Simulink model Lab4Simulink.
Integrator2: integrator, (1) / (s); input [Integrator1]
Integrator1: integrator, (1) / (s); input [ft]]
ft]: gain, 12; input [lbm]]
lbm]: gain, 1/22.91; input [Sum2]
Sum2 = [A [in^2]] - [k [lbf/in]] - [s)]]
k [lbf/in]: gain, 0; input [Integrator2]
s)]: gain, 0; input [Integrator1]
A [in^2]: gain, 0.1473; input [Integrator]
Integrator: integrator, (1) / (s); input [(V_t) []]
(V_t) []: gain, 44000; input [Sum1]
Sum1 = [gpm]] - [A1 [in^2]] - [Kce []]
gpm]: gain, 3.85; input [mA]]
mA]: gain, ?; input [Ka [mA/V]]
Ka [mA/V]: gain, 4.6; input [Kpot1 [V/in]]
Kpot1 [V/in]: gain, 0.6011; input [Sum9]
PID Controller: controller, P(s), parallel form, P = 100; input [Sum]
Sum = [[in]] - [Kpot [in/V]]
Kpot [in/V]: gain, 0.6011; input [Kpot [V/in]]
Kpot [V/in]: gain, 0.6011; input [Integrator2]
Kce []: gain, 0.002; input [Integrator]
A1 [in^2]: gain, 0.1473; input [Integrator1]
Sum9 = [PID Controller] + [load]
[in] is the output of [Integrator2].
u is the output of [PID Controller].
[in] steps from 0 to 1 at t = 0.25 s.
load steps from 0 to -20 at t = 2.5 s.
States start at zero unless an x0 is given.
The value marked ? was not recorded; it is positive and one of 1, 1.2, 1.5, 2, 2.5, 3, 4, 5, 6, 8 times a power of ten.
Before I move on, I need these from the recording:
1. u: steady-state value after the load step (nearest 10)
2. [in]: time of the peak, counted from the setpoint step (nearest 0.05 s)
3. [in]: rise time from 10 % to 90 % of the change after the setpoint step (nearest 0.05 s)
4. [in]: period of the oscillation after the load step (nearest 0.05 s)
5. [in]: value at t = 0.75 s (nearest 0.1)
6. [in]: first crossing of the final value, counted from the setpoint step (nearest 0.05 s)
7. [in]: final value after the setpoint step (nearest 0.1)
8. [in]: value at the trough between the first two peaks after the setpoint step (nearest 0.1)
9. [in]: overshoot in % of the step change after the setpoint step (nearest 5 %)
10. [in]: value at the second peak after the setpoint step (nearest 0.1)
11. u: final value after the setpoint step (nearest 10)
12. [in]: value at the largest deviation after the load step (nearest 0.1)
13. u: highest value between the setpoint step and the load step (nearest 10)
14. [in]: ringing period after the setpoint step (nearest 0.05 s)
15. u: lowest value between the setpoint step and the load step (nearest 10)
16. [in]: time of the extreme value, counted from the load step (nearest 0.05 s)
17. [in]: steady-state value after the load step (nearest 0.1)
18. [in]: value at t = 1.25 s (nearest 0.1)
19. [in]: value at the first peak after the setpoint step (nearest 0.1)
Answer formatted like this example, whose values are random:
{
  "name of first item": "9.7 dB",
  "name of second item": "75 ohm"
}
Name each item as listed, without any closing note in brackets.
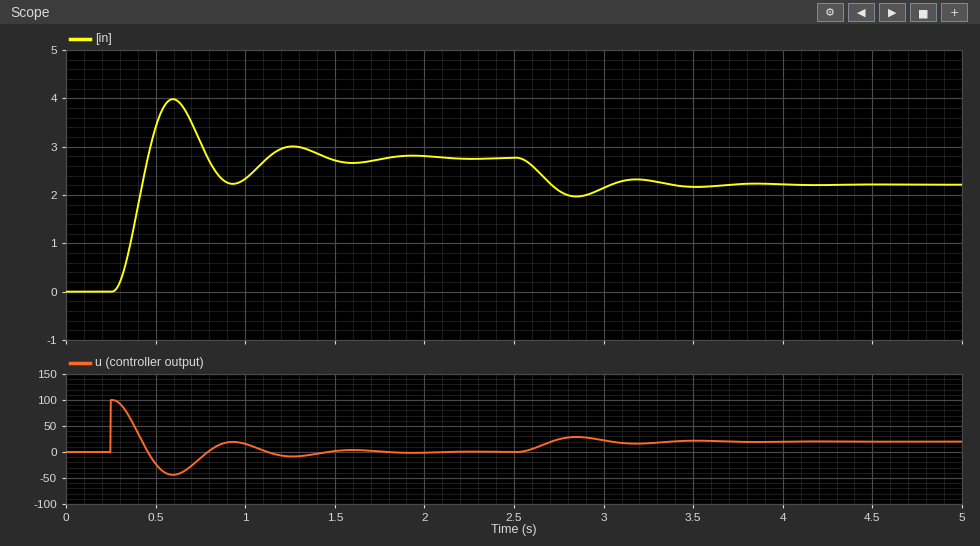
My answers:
{
  "u: steady-state value after the load step": "20",
  "[in]: time of the peak, counted from the setpoint step": "0.35 s",
  "[in]: rise time from 10 % to 90 % of the change after the setpoint step": "0.15 s",
  "[in]: period of the oscillation after the load step": "0.65 s",
  "[in]: value at t = 0.75 s": "3.1",
  "[in]: first crossing of the final value, counted from the setpoint step": "0.20 s",
  "[in]: final value after the setpoint step": "2.8",
  "[in]: value at the trough between the first two peaks after the setpoint step": "2.2",
  "[in]: overshoot in % of the step change after the setpoint step": "45 %",
  "[in]: value at the second peak after the setpoint step": "3.0",
  "u: final value after the setpoint step": "0",
  "[in]: value at the largest deviation after the load step": "2.0",
  "u: highest value between the setpoint step and the load step": "100",
  "[in]: ringing period after the setpoint step": "0.65 s",
  "u: lowest value between the setpoint step and the load step": "-40",
  "[in]: time of the extreme value, counted from the load step": "0.35 s",
  "[in]: steady-state value after the load step": "2.2",
  "[in]: value at t = 1.25 s": "3.0",
  "[in]: value at the first peak after the setpoint step": "4.0"
}
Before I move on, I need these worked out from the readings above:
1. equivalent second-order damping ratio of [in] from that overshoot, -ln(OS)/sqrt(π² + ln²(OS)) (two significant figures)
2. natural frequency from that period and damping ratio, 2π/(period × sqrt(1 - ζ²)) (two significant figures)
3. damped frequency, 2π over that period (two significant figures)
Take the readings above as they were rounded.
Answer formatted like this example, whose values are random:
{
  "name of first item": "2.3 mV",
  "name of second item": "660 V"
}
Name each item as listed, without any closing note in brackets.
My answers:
{
  "equivalent second-order damping ratio of [in] from that overshoot, -ln(OS)/sqrt(π² + ln²(OS))": "0.25",
  "natural frequency from that period and damping ratio, 2π/(period × sqrt(1 - ζ²))": "10.0 rad/s",
  "damped frequency, 2π over that period": "9.7 rad/s"
}
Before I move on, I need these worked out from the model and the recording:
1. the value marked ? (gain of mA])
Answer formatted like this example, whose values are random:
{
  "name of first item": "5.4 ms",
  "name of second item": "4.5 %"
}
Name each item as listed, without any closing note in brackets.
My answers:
{
  "the value marked ?": "0.006"
}
